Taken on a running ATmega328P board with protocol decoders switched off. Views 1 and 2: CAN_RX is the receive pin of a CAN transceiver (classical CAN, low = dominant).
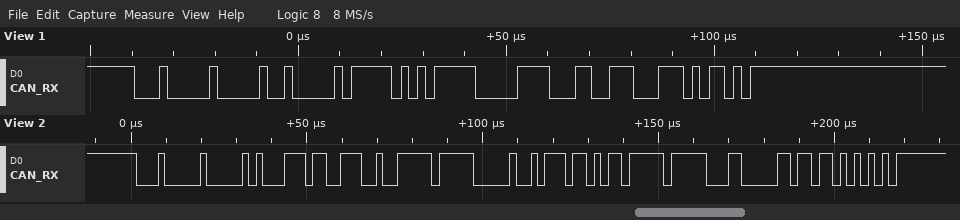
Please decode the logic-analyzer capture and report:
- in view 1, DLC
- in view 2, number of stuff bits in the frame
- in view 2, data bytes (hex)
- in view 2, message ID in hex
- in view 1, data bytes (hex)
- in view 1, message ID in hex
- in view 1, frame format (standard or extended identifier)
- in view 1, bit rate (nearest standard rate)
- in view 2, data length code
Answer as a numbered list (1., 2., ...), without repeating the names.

1. 4
2. 8
3. EC E4 FF C0 BB 5B FF 30
4. 0x100
5. 0F D7 C3 8C
6. 0x100
7. standard
8. 500 kbit/s
9. 8
